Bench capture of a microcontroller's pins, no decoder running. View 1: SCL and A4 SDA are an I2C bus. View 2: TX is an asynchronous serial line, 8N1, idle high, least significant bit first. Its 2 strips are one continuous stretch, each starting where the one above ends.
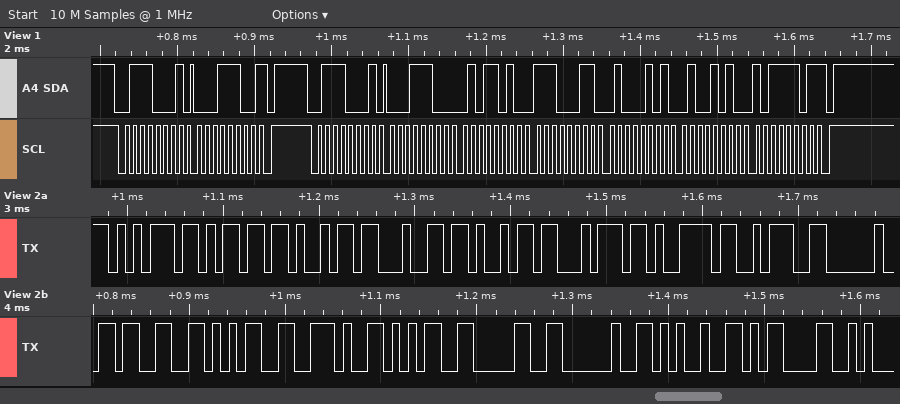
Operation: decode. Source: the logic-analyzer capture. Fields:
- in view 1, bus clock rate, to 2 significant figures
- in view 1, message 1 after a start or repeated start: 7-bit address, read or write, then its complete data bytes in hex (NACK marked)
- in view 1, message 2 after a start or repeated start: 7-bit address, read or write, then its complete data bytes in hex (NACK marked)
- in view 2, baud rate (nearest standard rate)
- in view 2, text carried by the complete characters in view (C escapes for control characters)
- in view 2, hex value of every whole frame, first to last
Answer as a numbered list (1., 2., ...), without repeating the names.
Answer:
1. 100 kHz
2. 0x38 read: 1C NACK
3. 0x38 read: 1C 5A E3 45 4A BD NACK
4. 115200 baud
5. "umidity: 35.50 %\r"
6. 0x75 0x6D 0x69 0x64 0x69 0x74 0x79 0x3A 0x20 0x33 0x35 0x2E 0x35 0x30 0x20 0x25 0x0D
